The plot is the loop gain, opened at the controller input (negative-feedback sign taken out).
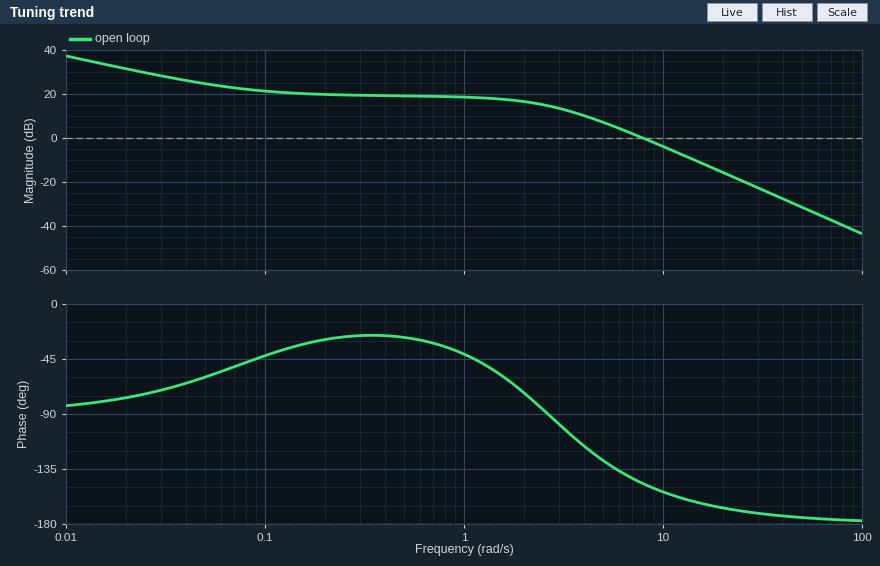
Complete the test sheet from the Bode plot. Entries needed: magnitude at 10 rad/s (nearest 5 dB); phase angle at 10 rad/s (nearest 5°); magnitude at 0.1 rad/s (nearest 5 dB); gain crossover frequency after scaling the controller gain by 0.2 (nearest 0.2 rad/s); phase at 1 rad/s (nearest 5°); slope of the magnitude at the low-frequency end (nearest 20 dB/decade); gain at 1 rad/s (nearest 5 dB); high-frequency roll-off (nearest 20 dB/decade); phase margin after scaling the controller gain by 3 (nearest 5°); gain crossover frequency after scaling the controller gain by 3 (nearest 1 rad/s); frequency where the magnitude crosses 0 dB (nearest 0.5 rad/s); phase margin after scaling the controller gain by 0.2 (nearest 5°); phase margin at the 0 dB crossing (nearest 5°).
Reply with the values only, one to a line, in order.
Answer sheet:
-5 dB
-155°
20 dB
2.8 rad/s
-40°
-20 dB/decade
20 dB
-40 dB/decade
20°
14 rad/s
8.0 rad/s
85°
35°
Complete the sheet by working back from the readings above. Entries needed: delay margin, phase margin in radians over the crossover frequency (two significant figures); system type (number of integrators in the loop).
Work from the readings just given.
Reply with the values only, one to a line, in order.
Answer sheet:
0.076 s
1
